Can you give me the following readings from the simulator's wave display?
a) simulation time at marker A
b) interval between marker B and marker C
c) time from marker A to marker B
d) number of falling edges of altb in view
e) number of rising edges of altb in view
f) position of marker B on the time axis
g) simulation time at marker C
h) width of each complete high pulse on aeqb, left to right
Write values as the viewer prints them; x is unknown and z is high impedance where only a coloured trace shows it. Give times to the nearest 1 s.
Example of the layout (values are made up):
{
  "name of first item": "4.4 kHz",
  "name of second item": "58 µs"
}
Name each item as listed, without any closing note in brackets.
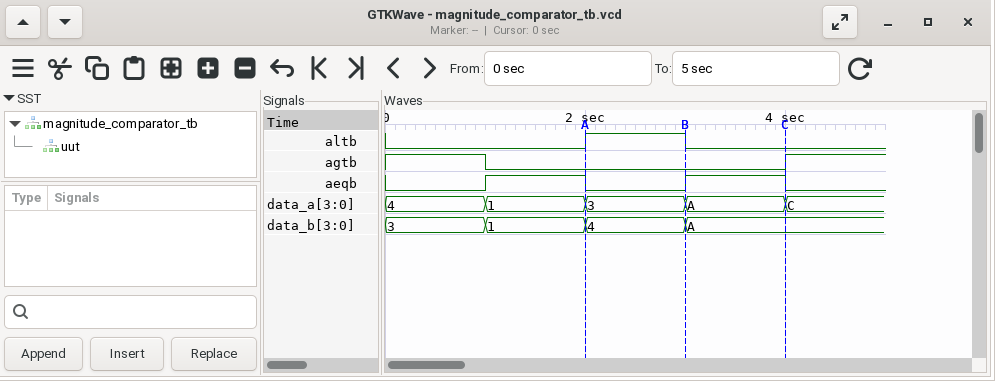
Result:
{
  "simulation time at marker A": "2 s",
  "interval between marker B and marker C": "1 s",
  "time from marker A to marker B": "1 s",
  "number of falling edges of altb in view": "1",
  "number of rising edges of altb in view": "1",
  "position of marker B on the time axis": "3 s",
  "simulation time at marker C": "4 s",
  "width of each complete high pulse on aeqb, left to right": "1 s, 1 s"
}
